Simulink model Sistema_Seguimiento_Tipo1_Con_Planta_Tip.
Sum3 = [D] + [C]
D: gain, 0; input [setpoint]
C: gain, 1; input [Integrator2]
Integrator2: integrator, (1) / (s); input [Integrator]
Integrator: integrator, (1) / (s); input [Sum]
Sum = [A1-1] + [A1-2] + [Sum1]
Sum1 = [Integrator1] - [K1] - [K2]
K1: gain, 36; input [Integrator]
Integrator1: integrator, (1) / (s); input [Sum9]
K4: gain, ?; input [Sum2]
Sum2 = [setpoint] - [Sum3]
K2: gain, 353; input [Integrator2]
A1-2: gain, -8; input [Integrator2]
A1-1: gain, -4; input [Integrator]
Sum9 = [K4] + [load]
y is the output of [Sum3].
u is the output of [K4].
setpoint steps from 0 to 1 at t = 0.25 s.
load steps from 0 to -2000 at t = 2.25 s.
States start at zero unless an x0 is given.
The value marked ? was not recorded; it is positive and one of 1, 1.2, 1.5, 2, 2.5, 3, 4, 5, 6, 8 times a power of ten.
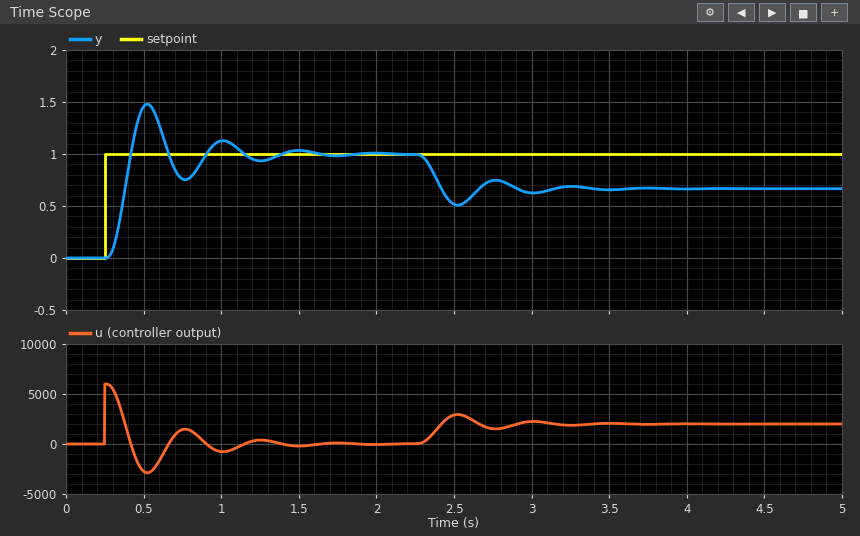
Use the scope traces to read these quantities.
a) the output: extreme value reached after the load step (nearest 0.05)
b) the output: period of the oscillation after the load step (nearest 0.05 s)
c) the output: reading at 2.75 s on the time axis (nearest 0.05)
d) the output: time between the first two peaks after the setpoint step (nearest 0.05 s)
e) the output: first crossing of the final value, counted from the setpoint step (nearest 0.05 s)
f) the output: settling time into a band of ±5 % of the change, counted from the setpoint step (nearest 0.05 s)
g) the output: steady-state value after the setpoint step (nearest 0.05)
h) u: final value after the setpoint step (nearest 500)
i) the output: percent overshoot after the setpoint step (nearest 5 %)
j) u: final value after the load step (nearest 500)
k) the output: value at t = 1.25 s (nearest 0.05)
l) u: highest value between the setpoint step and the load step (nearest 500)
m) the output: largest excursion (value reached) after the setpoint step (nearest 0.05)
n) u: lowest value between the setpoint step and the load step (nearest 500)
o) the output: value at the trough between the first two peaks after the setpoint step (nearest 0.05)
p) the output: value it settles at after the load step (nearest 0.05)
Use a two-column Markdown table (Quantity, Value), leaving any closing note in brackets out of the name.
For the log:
| Quantity | Value |
|---|---|
| the output: extreme value reached after the load step | 0.50 |
| the output: period of the oscillation after the load step | 0.50 s |
| the output: reading at 2.75 s on the time axis | 0.75 |
| the output: time between the first two peaks after the setpoint step | 0.50 s |
| the output: first crossing of the final value, counted from the setpoint step | 0.15 s |
| the output: settling time into a band of ±5 % of the change, counted from the setpoint step | 1.05 s |
| the output: steady-state value after the setpoint step | 1.00 |
| u: final value after the setpoint step | 0 |
| the output: percent overshoot after the setpoint step | 50 % |
| u: final value after the load step | 2000 |
| the output: value at t = 1.25 s | 0.95 |
| u: highest value between the setpoint step and the load step | 6000 |
| the output: largest excursion (value reached) after the setpoint step | 1.50 |
| u: lowest value between the setpoint step and the load step | -3000 |
| the output: value at the trough between the first two peaks after the setpoint step | 0.75 |
| the output: value it settles at after the load step | 0.65 |
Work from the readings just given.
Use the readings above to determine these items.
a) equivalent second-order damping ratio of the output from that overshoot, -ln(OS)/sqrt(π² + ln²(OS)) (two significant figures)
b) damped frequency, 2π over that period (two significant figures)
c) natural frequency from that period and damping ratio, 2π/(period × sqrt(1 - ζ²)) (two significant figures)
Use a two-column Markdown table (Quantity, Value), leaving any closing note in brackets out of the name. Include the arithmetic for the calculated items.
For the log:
| Quantity | Value |
|---|---|
| equivalent second-order damping ratio of the output from that overshoot, -ln(OS)/sqrt(π² + ln²(OS)) | ln(0.5) = -0.693; 0.693 / sqrt(9.870 + 0.480) = 0.22 |
| damped frequency, 2π over that period | 2π / 0.5 = 13 rad/s |
| natural frequency from that period and damping ratio, 2π/(period × sqrt(1 - ζ²)) | 2π / (0.5 × sqrt(1 - 0.22²)) = 13 rad/s |
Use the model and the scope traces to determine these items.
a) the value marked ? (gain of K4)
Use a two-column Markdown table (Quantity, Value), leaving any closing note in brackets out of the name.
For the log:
| Quantity | Value |
|---|---|
| the value marked ? | 6000 |
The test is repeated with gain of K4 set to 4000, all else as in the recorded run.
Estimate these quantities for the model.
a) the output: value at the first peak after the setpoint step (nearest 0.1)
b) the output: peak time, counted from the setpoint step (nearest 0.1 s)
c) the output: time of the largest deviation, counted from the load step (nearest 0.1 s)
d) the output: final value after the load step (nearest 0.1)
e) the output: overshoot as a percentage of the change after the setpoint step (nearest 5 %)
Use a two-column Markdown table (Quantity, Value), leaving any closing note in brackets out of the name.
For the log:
| Quantity | Value |
|---|---|
| the output: value at the first peak after the setpoint step | 1.3 |
| the output: peak time, counted from the setpoint step | 0.3 s |
| the output: time of the largest deviation, counted from the load step | 0.3 s |
| the output: final value after the load step | 0.5 |
| the output: overshoot as a percentage of the change after the setpoint step | 30 % |
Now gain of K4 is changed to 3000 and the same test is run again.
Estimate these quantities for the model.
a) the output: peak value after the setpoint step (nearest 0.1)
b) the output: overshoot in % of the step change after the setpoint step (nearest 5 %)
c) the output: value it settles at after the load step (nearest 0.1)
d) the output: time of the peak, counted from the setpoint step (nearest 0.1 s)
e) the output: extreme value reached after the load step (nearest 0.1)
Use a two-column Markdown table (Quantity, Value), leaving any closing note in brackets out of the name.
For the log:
| Quantity | Value |
|---|---|
| the output: peak value after the setpoint step | 1.2 |
| the output: overshoot in % of the step change after the setpoint step | 20 % |
| the output: value it settles at after the load step | 0.3 |
| the output: time of the peak, counted from the setpoint step | 0.4 s |
| the output: extreme value reached after the load step | 0.2 |
